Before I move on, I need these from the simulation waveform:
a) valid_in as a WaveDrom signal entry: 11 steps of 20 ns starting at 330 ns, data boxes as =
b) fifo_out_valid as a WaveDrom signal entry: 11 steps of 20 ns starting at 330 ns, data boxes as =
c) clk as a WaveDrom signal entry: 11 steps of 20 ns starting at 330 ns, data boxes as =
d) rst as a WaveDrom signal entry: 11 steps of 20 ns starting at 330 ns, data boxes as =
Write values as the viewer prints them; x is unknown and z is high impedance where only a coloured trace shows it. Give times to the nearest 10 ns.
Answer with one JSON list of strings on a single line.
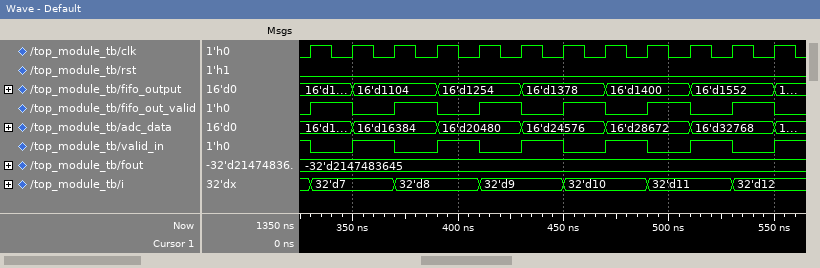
["{name: 'valid_in', wave: '01010101010'}", "{name: 'fifo_out_valid', wave: '10101010101'}", "{name: 'clk', wave: 'p..........'}", "{name: 'rst', wave: '0..........'}"]
